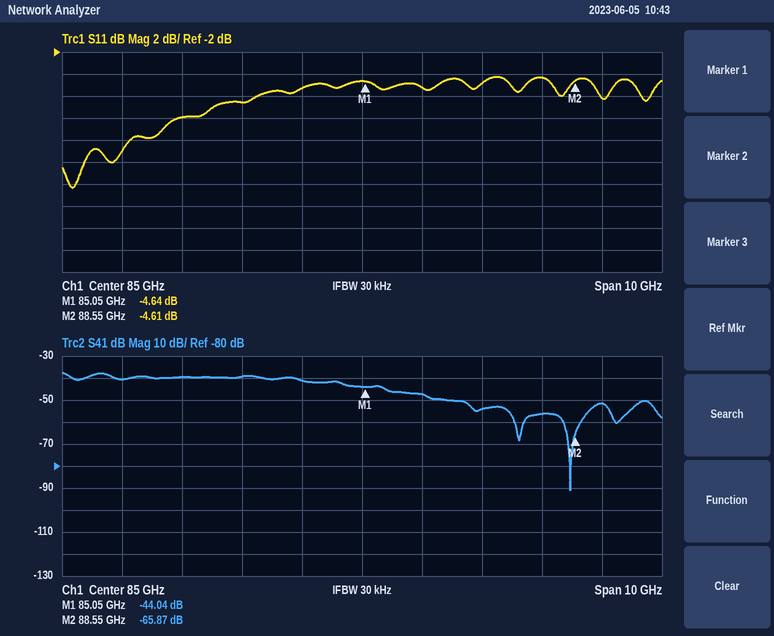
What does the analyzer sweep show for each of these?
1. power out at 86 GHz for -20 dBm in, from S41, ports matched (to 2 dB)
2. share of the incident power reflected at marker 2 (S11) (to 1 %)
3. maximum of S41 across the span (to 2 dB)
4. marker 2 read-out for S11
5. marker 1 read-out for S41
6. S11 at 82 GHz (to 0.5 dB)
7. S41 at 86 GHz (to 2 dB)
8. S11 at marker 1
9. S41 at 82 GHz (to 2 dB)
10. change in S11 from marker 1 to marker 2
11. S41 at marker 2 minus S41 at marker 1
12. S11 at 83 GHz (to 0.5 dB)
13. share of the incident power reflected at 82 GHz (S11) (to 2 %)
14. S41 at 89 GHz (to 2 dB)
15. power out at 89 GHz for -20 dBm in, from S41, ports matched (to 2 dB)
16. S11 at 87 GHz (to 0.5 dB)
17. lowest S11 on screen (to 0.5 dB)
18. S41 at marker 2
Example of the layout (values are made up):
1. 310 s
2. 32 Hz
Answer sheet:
1. -68 dBm
2. 35 %
3. -38 dB
4. -4.61 dB
5. -44.04 dB
6. -8.0 dB
7. -48 dB
8. -4.64 dB
9. -40 dB
10. 0.03 dB
11. -21.83 dB
12. -6.5 dB
13. 16 %
14. -52 dB
15. -72 dBm
16. -5.0 dB
17. -14.5 dB
18. -65.87 dB
